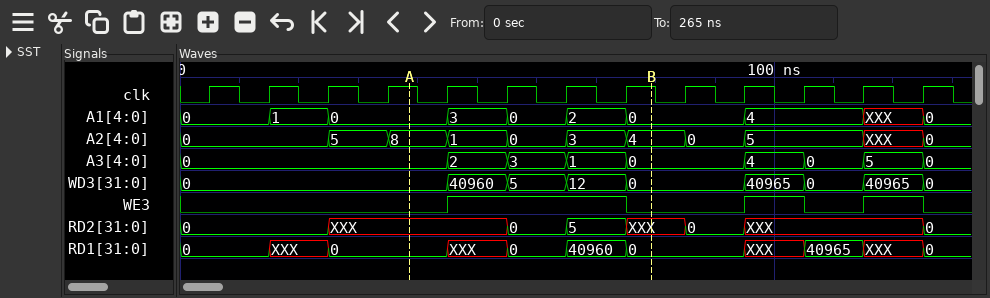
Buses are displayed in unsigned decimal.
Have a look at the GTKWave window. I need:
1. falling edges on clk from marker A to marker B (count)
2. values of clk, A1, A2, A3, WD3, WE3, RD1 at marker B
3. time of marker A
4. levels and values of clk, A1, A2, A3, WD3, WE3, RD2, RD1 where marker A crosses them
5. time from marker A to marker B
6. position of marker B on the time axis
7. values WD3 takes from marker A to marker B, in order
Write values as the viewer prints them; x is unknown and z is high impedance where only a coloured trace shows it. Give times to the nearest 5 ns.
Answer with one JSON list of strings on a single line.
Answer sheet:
["4", "clk=1, A1=0, A2=4, A3=0, WD3=0, WE3=0, RD1=0", "40 ns", "clk=1, A1=0, A2=8, A3=0, WD3=0, WE3=0, RD2=XXX, RD1=0", "40 ns", "80 ns", "0, 40960, 5, 12, 0"]
